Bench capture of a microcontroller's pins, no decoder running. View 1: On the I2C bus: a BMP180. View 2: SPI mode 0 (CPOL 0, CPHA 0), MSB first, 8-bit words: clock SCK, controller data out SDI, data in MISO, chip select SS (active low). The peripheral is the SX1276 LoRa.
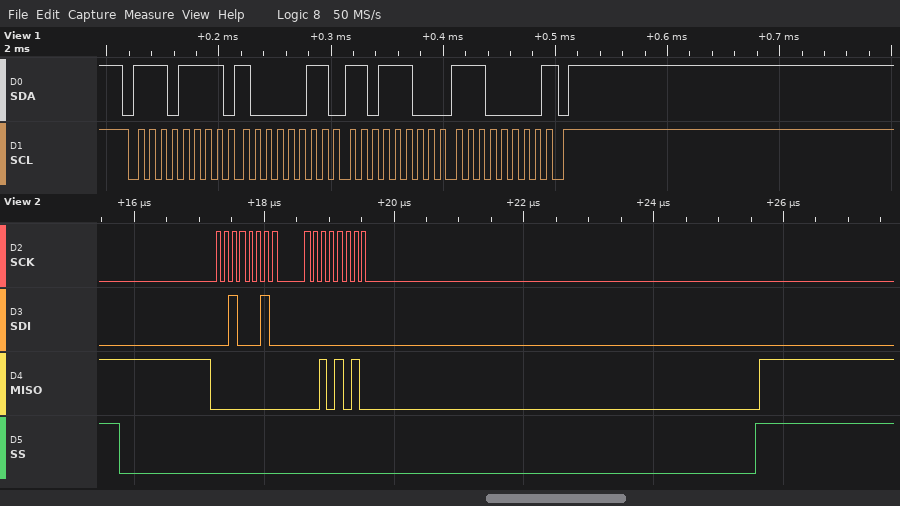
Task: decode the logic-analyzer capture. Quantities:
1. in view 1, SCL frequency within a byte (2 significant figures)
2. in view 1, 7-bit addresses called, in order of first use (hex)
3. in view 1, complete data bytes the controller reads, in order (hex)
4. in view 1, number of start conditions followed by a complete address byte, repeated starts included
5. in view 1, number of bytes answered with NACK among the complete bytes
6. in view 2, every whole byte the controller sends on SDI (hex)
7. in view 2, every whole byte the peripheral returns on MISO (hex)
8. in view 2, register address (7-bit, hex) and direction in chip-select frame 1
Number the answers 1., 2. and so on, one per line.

1. 100 kHz
2. 0x77
3. 83 DC E0
4. 1
5. 1
6. 0x22 0x00
7. 0x00 0x2A
8. 0x22 read
